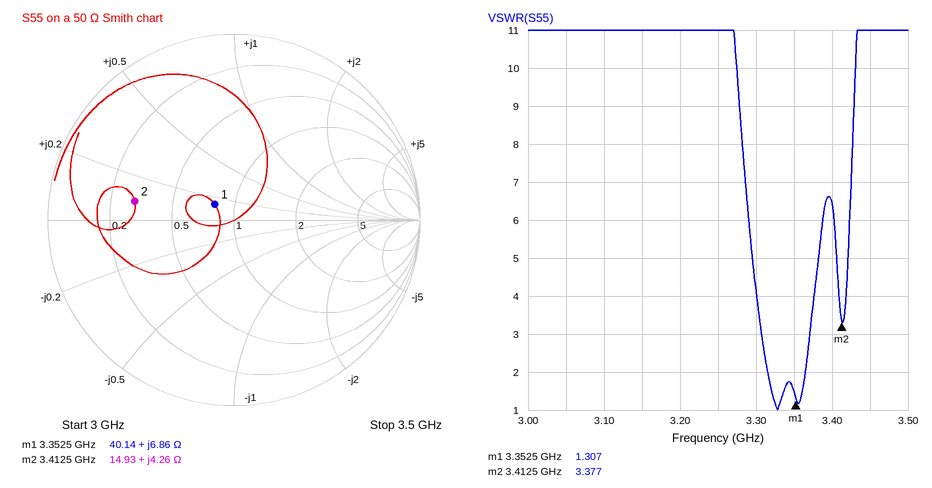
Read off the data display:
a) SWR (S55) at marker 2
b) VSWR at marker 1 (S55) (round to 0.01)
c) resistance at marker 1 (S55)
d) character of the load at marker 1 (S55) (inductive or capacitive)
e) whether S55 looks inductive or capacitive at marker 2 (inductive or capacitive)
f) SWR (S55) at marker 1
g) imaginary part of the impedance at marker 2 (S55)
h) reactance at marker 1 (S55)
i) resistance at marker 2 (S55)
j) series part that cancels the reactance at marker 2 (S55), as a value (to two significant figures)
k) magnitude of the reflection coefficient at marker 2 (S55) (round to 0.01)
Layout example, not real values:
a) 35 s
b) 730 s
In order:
a) 3.377
b) 1.31
c) 40.14 Ω
d) inductive
e) inductive
f) 1.307
g) +4.26 Ω
h) +6.86 Ω
i) 14.93 Ω
j) 11 pF
k) 0.54
